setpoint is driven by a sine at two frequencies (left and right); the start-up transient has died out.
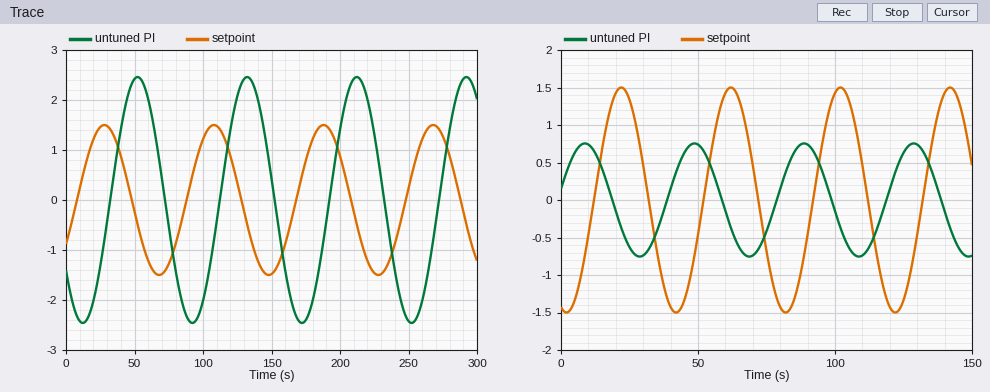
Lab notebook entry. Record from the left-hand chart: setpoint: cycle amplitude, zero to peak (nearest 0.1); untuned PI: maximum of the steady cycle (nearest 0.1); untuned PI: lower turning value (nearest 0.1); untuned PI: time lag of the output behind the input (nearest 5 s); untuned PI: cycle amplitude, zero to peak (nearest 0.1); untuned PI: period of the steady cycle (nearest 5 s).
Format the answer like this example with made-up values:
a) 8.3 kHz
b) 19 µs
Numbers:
a) 1.5
b) 2.5
c) -2.5
d) 25 s
e) 2.5
f) 80 s
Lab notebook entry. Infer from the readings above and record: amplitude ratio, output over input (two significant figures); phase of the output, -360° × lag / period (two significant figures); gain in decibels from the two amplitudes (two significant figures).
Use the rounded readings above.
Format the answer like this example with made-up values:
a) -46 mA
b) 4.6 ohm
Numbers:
a) 1.7
b) -110°
c) 4.4 dB
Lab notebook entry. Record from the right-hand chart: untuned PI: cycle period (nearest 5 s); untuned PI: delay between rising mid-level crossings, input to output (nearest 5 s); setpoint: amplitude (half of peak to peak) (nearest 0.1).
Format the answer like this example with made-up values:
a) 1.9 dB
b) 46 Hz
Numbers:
a) 40 s
b) 25 s
c) 1.5
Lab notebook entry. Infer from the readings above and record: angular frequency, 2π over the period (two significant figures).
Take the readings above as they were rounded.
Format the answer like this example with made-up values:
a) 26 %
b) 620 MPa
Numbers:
a) 0.16 rad/s
